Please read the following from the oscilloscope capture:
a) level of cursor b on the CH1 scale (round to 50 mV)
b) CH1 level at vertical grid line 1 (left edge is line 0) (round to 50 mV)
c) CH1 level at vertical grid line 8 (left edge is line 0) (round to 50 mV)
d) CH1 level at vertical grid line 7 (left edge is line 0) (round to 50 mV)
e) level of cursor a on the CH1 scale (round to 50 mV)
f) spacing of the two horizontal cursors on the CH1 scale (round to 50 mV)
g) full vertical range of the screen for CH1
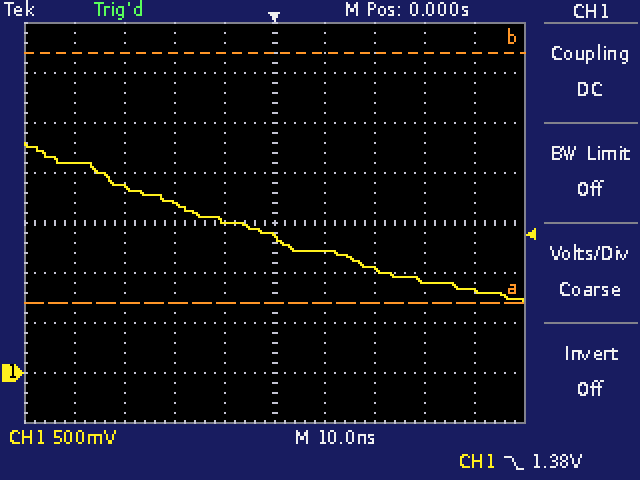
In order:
3.20 V
2.10 V
900 mV
1.05 V
700 mV
2.50 V
4 V
